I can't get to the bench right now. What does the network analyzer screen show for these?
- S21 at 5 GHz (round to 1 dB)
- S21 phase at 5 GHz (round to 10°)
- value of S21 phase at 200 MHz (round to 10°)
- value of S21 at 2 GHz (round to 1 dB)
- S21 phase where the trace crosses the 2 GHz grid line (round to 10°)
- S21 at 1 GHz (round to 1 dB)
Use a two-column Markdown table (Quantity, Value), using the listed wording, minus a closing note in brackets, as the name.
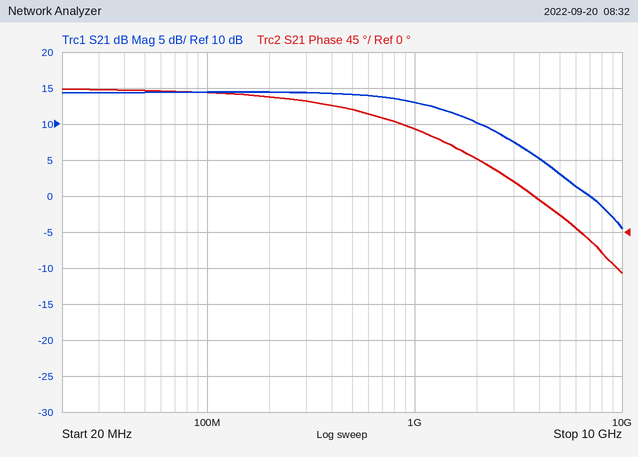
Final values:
| Quantity | Value |
|---|---|
| S21 at 5 GHz | 3 dB |
| S21 phase at 5 GHz | 20° |
| value of S21 phase at 200 MHz | 170° |
| value of S21 at 2 GHz | 10 dB |
| S21 phase where the trace crosses the 2 GHz grid line | 90° |
| S21 at 1 GHz | 13 dB |
